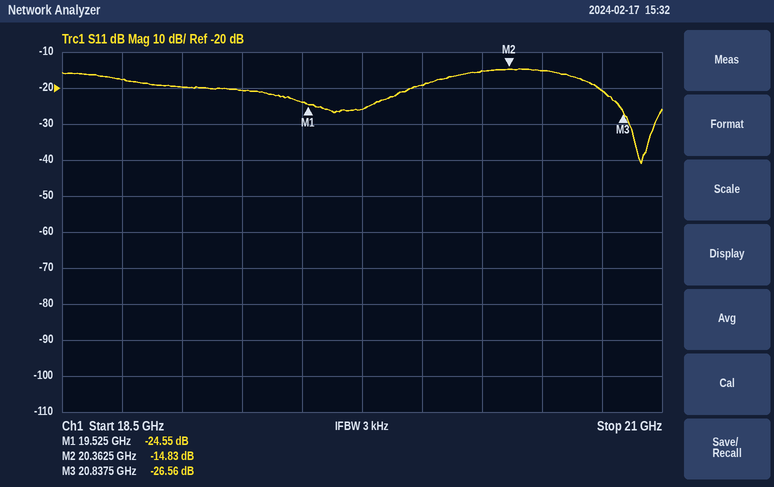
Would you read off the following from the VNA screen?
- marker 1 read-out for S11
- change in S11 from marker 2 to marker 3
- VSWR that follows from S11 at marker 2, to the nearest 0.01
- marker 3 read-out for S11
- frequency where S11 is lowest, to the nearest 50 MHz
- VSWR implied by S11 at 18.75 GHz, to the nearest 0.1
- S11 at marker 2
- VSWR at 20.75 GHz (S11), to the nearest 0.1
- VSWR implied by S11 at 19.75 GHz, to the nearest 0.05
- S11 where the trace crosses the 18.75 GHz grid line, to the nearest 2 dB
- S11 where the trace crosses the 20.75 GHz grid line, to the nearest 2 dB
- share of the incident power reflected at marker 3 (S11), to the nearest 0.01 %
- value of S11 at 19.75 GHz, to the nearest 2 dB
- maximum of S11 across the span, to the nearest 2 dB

-24.55 dB
-11.73 dB
1.44
-26.56 dB
20.90 GHz
1.3
-14.83 dB
1.2
1.10
-18 dB
-20 dB
0.22 %
-26 dB
-14 dB
